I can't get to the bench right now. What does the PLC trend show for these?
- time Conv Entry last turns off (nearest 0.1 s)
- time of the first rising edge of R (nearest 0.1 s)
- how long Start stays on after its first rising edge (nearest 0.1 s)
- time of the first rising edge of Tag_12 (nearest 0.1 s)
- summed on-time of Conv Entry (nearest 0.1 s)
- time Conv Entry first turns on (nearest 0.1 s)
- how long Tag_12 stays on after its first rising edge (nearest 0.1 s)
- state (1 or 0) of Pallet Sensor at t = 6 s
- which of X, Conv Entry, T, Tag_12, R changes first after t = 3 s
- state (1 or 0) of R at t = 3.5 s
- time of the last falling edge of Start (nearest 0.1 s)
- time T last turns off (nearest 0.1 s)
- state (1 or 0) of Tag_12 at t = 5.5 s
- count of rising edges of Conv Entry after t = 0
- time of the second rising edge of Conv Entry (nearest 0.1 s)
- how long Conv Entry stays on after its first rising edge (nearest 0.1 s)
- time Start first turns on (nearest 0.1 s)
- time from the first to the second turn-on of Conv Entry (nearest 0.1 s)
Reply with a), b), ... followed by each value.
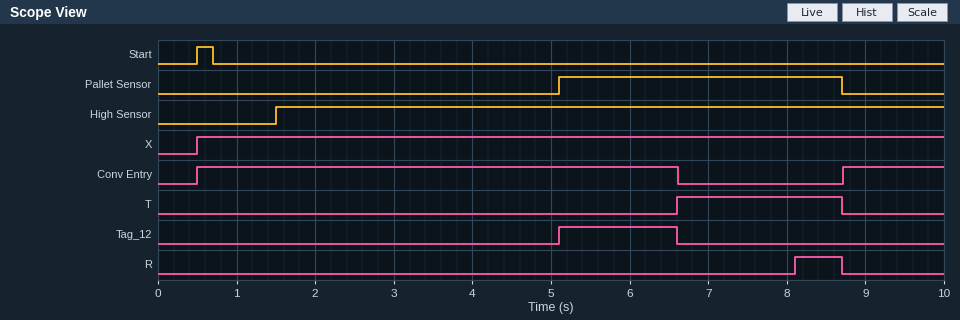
a) 6.6 s
b) 8.1 s
c) 0.2 s
d) 5.1 s
e) 7.4 s
f) 0.5 s
g) 1.5 s
h) 1
i) Tag_12
j) 0
k) 0.7 s
l) 8.7 s
m) 1
n) 2
o) 8.7 s
p) 6.1 s
q) 0.5 s
r) 8.2 s
